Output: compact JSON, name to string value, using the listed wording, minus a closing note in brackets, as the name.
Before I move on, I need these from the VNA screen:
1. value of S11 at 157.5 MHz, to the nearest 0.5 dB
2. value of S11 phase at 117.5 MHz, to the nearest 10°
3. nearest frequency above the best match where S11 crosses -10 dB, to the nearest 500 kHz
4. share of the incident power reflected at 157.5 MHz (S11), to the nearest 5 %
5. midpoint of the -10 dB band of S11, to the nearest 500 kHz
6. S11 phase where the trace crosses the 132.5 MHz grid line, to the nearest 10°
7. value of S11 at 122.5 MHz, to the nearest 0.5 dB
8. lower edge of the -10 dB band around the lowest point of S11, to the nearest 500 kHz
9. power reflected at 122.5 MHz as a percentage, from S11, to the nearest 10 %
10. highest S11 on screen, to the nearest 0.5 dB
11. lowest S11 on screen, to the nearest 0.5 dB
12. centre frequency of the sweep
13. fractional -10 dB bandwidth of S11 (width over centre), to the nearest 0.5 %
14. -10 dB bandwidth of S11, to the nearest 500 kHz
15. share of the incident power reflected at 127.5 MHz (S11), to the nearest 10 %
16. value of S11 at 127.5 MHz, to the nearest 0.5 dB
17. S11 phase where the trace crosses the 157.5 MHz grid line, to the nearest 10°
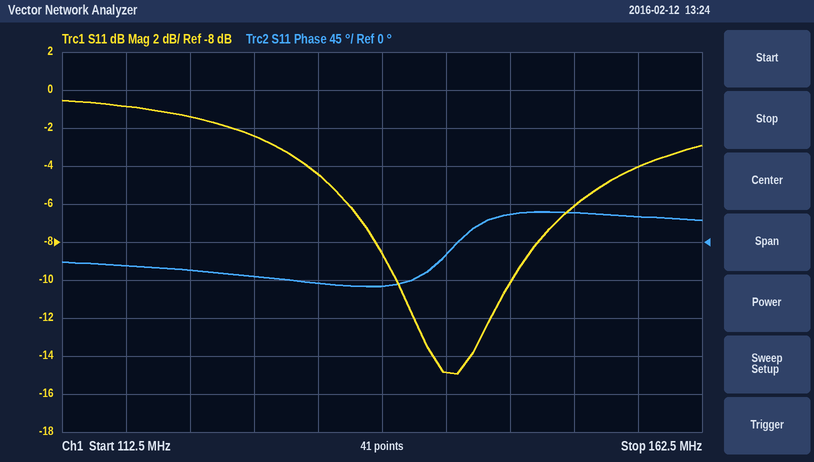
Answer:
{"value of S11 at 157.5 MHz, to the nearest 0.5 dB": "-4.0 dB", "value of S11 phase at 117.5 MHz, to the nearest 10°": "-30°", "nearest frequency above the best match where S11 crosses -10 dB, to the nearest 500 kHz": "147.5 MHz", "share of the incident power reflected at 157.5 MHz (S11), to the nearest 5 %": "40 %", "midpoint of the -10 dB band of S11, to the nearest 500 kHz": "143.0 MHz", "S11 phase where the trace crosses the 132.5 MHz grid line, to the nearest 10°": "-50°", "value of S11 at 122.5 MHz, to the nearest 0.5 dB": "-1.5 dB", "lower edge of the -10 dB band around the lowest point of S11, to the nearest 500 kHz": "138.5 MHz", "power reflected at 122.5 MHz as a percentage, from S11, to the nearest 10 %": "70 %", "highest S11 on screen, to the nearest 0.5 dB": "-0.5 dB", "lowest S11 on screen, to the nearest 0.5 dB": "-15.0 dB", "centre frequency of the sweep": "137.5 MHz", "fractional -10 dB bandwidth of S11 (width over centre), to the nearest 0.5 %": "6.5 %", "-10 dB bandwidth of S11, to the nearest 500 kHz": "9.0 MHz", "share of the incident power reflected at 127.5 MHz (S11), to the nearest 10 %": "60 %", "value of S11 at 127.5 MHz, to the nearest 0.5 dB": "-2.5 dB", "S11 phase where the trace crosses the 157.5 MHz grid line, to the nearest 10°": "30°"}
